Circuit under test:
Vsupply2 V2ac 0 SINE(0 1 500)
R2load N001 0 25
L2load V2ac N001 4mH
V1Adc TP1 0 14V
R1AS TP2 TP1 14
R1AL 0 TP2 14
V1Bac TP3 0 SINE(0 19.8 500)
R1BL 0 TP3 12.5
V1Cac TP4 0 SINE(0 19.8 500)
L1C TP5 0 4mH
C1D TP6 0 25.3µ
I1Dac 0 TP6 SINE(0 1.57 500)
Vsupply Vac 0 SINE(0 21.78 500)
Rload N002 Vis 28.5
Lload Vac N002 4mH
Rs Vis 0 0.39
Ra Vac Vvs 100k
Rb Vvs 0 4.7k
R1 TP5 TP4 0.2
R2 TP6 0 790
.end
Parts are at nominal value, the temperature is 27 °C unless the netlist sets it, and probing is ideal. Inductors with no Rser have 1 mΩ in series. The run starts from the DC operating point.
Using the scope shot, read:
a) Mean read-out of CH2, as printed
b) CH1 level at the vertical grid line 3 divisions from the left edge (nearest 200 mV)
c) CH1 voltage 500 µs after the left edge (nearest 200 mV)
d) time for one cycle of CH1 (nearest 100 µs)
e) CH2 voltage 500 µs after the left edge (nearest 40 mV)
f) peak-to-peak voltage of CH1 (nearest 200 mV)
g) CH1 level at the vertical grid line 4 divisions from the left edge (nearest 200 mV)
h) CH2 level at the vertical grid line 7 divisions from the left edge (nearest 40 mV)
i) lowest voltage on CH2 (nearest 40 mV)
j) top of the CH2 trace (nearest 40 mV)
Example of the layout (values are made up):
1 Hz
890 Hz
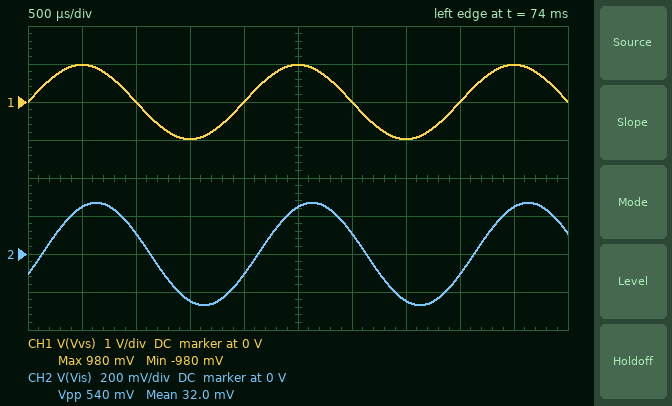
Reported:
32.0 mV
-1.0 V
1.0 V
2.0 ms
240 mV
2.0 V
0 V
-240 mV
-280 mV
280 mV
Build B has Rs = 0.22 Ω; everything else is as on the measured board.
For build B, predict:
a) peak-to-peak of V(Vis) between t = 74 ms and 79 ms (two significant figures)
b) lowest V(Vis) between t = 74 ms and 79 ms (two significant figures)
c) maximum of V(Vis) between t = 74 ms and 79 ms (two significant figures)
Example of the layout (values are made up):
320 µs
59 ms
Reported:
310 mV
-150 mV
150 mV
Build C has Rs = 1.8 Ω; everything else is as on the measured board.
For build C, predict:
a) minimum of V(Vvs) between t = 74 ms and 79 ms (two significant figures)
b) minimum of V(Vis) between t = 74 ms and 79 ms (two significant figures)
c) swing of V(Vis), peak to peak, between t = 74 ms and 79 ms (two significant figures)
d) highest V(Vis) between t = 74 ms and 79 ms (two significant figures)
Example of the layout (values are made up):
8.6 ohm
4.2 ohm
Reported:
-980 mV
-1.2 V
2.4 V
1.2 V
